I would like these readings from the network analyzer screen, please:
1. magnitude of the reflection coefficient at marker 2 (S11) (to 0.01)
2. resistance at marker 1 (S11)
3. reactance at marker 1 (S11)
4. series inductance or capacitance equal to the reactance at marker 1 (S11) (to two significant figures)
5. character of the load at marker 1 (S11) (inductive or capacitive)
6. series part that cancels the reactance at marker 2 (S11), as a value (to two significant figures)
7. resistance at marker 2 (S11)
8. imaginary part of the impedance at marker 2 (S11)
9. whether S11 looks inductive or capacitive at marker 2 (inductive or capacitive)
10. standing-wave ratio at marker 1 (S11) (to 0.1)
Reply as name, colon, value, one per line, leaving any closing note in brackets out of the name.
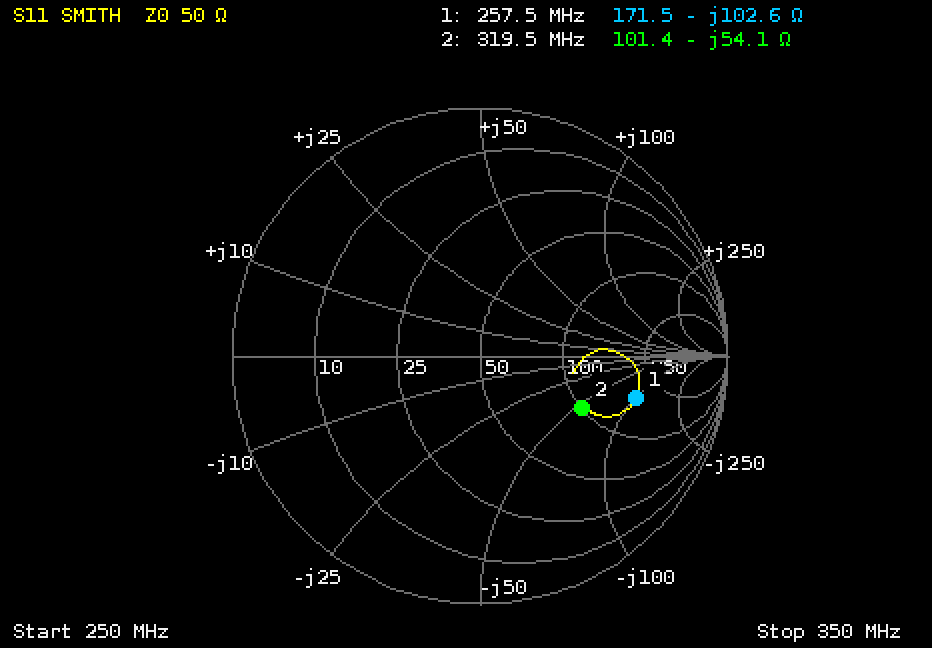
magnitude of the reflection coefficient at marker 2 (S11): 0.46
resistance at marker 1: 171.5 Ω
reactance at marker 1: -102.6 Ω
series inductance or capacitance equal to the reactance at marker 1 (S11): 6.0 pF
character of the load at marker 1 (S11): capacitive
series part that cancels the reactance at marker 2 (S11), as a value: 27 nH
resistance at marker 2: 101.4 Ω
imaginary part of the impedance at marker 2: -54.1 Ω
whether S11 looks inductive or capacitive at marker 2: capacitive
standing-wave ratio at marker 1 (S11): 4.7
